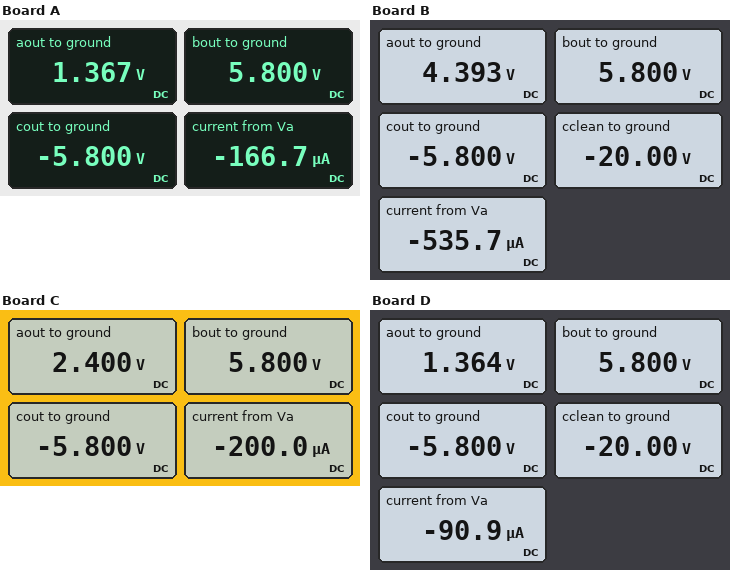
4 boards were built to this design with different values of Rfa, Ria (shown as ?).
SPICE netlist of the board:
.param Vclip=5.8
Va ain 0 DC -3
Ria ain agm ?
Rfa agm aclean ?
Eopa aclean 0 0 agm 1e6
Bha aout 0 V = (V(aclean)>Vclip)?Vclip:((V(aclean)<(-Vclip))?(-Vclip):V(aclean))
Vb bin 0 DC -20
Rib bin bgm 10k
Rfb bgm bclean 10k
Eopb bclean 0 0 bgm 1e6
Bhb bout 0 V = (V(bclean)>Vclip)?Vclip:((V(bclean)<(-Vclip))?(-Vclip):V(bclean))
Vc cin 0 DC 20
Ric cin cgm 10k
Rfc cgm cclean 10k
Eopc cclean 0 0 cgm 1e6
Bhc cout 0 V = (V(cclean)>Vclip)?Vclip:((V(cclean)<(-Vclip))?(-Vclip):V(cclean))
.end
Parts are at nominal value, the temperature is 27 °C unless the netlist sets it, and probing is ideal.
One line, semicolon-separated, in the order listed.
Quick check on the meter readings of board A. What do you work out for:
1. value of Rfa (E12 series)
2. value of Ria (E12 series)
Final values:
8.2 kΩ; 18 kΩ
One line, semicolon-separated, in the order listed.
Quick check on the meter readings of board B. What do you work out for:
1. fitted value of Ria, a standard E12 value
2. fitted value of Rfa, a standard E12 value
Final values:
5.6 kΩ; 8.2 kΩ
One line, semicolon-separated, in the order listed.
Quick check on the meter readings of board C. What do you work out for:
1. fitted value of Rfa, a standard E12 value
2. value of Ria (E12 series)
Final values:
12 kΩ; 15 kΩ
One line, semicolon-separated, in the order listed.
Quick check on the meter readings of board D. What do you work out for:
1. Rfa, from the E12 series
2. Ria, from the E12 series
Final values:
15 kΩ; 33 kΩ
